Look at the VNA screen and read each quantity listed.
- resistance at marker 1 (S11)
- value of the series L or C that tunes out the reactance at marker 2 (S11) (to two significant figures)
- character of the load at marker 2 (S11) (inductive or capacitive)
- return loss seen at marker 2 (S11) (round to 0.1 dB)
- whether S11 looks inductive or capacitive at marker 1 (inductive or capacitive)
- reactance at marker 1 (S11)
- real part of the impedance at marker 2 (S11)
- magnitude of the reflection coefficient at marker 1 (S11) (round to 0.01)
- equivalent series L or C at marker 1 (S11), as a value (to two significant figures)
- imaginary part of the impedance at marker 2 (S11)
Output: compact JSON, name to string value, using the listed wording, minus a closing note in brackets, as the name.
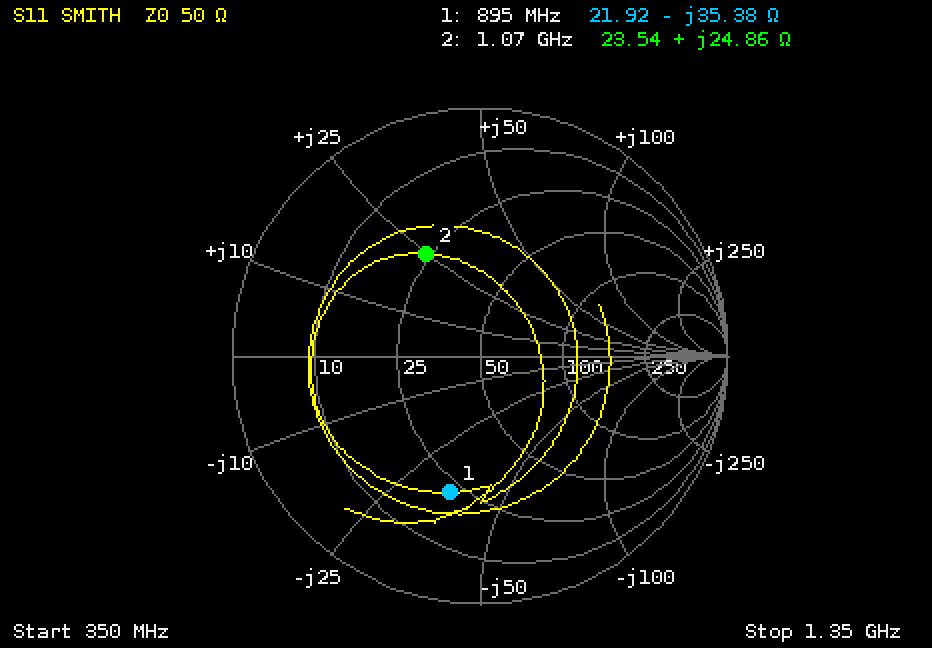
{"resistance at marker 1": "21.92 Ω", "value of the series L or C that tunes out the reactance at marker 2 (S11)": "6.0 pF", "character of the load at marker 2 (S11)": "inductive", "return loss seen at marker 2 (S11)": "6.6 dB", "whether S11 looks inductive or capacitive at marker 1": "capacitive", "reactance at marker 1": "-35.38 Ω", "real part of the impedance at marker 2": "23.54 Ω", "magnitude of the reflection coefficient at marker 1 (S11)": "0.56", "equivalent series L or C at marker 1 (S11), as a value": "5.0 pF", "imaginary part of the impedance at marker 2": "+24.86 Ω"}
